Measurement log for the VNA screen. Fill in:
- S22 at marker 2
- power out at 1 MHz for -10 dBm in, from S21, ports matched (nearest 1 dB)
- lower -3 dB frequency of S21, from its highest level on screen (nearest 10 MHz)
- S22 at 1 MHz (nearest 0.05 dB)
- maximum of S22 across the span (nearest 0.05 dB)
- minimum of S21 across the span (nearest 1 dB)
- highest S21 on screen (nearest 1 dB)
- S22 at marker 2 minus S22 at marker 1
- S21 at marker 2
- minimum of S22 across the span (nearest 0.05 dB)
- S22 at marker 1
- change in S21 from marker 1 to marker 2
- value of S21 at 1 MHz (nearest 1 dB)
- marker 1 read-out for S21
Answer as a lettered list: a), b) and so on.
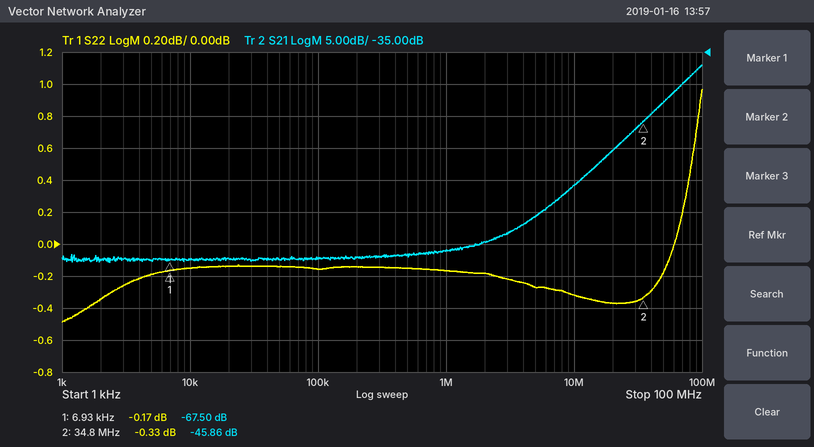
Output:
a) -0.33 dB
b) -76 dBm
c) 70 MHz
d) -0.15 dB
e) 0.95 dB
f) -68 dB
g) -37 dB
h) -0.16 dB
i) -45.86 dB
j) -0.50 dB
k) -0.17 dB
l) 21.64 dB
m) -66 dB
n) -67.50 dB
